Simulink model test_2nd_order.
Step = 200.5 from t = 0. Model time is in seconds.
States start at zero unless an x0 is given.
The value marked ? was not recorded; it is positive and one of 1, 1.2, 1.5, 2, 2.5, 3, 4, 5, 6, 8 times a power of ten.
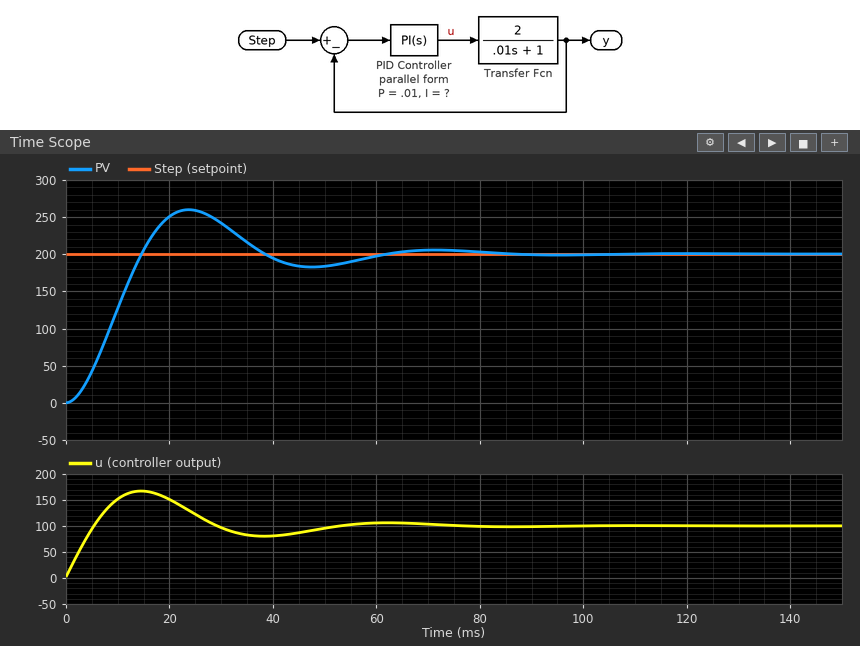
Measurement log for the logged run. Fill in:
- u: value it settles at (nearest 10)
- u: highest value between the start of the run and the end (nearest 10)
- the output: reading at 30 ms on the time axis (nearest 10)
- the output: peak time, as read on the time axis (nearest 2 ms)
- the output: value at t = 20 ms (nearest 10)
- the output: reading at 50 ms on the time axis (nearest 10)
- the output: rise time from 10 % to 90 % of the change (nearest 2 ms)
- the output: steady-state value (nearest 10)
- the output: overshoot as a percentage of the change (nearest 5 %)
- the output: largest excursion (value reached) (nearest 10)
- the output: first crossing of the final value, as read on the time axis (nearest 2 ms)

100
170
240
24 ms
250
180
10 ms
200
30 %
260
14 ms
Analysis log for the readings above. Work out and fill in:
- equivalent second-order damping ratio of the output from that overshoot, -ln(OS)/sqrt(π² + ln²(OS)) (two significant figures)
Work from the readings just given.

0.36
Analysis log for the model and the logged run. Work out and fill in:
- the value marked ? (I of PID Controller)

100
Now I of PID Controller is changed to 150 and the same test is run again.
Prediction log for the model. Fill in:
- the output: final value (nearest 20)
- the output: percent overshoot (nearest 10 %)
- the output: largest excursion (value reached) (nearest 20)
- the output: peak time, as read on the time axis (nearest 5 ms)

200
40 %
280
20 ms
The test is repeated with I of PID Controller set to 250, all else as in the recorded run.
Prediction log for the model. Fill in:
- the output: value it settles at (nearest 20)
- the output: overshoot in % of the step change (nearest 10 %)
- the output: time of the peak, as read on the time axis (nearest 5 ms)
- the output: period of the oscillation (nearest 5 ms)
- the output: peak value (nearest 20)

200
50 %
15 ms
30 ms
300
